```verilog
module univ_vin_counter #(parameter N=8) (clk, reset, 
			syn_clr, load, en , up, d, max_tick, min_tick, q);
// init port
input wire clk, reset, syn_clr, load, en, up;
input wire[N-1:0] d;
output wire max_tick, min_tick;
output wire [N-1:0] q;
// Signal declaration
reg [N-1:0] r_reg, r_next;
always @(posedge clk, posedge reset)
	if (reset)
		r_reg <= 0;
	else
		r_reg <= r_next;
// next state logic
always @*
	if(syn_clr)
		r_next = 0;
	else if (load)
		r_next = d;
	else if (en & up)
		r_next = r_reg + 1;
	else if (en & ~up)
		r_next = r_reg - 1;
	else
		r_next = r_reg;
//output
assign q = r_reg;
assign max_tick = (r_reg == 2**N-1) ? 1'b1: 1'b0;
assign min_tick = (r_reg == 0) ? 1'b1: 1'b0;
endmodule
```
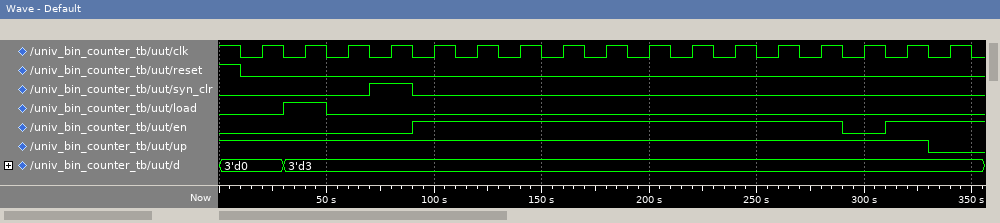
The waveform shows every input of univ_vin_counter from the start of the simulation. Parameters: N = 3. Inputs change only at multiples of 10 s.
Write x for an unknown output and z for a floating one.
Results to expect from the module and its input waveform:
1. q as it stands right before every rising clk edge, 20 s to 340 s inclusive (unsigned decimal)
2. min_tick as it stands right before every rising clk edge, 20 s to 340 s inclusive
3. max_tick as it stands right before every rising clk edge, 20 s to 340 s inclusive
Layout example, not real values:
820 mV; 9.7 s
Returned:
0, 0, 3, 3, 0, 1, 2, 3, 4, 5, 6, 7, 0, 1, 2, 2, 3; 1 1 0 0 1 0 0 0 0 0 0 0 1 0 0 0 0; 0 0 0 0 0 0 0 0 0 0 0 1 0 0 0 0 0
